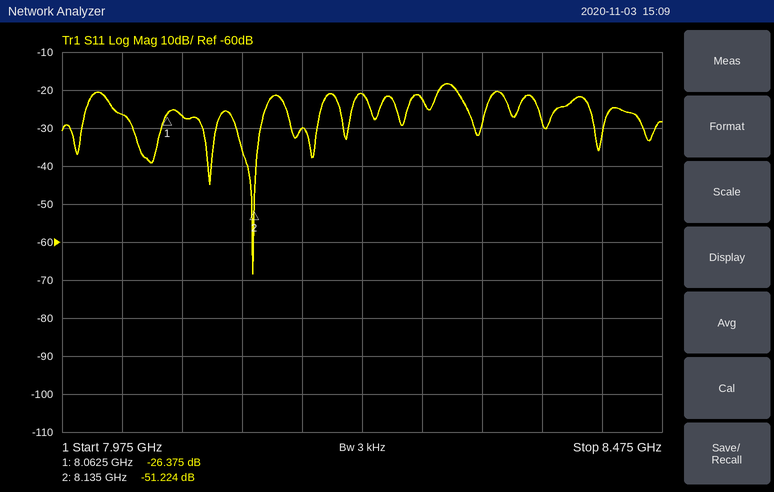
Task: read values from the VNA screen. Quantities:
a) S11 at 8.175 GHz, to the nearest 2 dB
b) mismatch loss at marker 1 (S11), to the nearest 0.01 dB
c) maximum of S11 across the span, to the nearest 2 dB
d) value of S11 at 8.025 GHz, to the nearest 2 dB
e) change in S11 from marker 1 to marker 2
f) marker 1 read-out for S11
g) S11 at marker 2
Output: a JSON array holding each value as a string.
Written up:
["-30 dB", "0.01 dB", "-18 dB", "-26 dB", "-24.849 dB", "-26.375 dB", "-51.224 dB"]
